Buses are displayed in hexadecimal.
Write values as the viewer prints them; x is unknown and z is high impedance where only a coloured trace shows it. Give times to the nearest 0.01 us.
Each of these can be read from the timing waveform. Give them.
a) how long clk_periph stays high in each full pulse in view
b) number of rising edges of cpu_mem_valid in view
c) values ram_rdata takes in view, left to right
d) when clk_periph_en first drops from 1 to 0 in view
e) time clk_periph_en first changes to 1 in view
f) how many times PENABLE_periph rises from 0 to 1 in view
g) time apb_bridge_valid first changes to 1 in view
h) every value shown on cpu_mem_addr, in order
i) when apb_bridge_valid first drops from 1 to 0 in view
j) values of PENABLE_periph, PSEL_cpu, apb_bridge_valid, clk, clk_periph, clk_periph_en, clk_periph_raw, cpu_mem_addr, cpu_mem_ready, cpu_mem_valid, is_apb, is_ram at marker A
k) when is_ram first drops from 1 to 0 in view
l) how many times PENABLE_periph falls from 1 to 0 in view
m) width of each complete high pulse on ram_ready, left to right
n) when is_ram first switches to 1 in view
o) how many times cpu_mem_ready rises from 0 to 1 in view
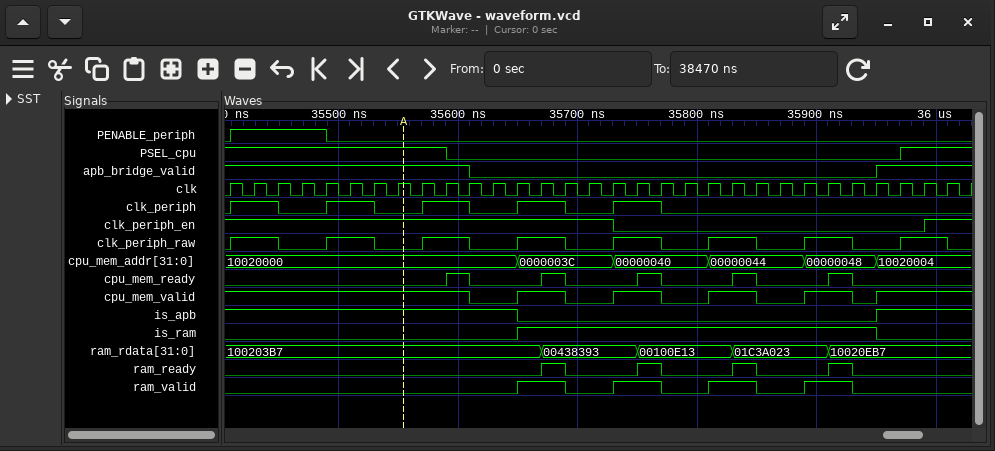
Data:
0.04 us, 0.04 us, 0.04 us, 0.04 us, 0.04 us
5
100203B7, 00438393, 00100E13, 01C3A023, 10020EB7
35.73 us
35.99 us
1
35.95 us
10020000, 0000003C, 00000040, 00000044, 00000048, 10020004
35.61 us
PENABLE_periph=0, PSEL_cpu=1, apb_bridge_valid=1, clk=1, clk_periph=0, clk_periph_en=1, clk_periph_raw=0, cpu_mem_addr=10020000, cpu_mem_ready=0, cpu_mem_valid=1, is_apb=1, is_ram=0
35.95 us
1
0.02 us, 0.02 us, 0.02 us, 0.02 us
35.65 us
5
